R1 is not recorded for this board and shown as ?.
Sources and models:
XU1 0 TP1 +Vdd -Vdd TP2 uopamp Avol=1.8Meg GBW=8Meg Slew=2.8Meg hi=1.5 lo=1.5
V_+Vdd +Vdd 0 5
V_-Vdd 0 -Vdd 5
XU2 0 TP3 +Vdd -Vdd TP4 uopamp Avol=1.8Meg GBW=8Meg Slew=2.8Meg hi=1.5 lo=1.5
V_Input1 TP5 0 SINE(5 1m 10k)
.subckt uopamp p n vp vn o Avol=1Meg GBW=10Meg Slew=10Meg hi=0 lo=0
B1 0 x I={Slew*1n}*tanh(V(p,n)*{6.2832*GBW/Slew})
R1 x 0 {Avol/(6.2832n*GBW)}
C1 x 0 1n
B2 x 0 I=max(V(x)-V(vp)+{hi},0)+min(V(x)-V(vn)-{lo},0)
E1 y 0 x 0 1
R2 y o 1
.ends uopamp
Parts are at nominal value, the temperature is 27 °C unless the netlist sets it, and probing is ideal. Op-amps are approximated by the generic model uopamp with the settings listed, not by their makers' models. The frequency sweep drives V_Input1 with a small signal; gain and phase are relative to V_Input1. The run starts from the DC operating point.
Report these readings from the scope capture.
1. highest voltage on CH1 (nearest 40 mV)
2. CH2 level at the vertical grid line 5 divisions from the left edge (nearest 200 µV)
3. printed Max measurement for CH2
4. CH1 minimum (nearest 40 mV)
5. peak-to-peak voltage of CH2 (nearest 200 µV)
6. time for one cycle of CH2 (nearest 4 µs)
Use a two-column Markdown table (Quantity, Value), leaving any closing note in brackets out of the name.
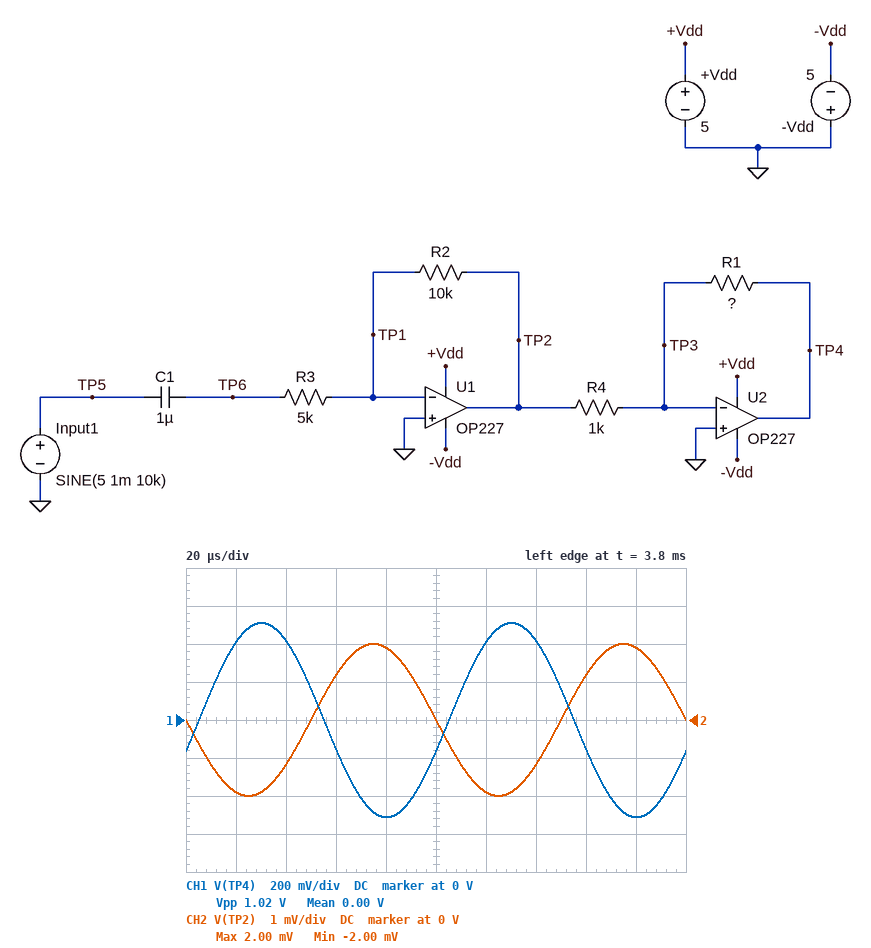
| Quantity | Value |
|---|---|
| highest voltage on CH1 | 520 mV |
| CH2 level at the vertical grid line 5 divisions from the left edge | 0 V |
| printed Max measurement for CH2 | 2.00 mV |
| CH1 minimum | -520 mV |
| peak-to-peak voltage of CH2 | 4.0 mV |
| time for one cycle of CH2 | 100 µs |
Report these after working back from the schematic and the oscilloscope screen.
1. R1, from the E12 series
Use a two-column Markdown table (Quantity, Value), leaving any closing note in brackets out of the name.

| Quantity | Value |
|---|---|
| R1, from the E12 series | 270 kΩ |
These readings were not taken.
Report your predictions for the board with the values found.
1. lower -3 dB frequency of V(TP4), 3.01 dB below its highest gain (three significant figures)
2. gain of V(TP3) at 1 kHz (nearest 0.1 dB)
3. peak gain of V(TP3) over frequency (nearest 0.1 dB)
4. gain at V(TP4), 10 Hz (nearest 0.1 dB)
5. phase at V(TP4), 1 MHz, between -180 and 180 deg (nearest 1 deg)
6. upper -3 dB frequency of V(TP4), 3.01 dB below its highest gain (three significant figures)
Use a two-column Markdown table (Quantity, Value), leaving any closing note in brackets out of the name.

| Quantity | Value |
|---|---|
| lower -3 dB frequency of V(TP4), 3.01 dB below its highest gain | 31.8 Hz |
| gain of V(TP3) at 1 kHz | -23.4 dB |
| peak gain of V(TP3) over frequency | 5.9 dB |
| gain at V(TP4), 10 Hz | 44.2 dB |
| phase at V(TP4), 1 MHz, between -180 and 180 deg | -109 deg |
| upper -3 dB frequency of V(TP4), 3.01 dB below its highest gain | 29.6 kHz |
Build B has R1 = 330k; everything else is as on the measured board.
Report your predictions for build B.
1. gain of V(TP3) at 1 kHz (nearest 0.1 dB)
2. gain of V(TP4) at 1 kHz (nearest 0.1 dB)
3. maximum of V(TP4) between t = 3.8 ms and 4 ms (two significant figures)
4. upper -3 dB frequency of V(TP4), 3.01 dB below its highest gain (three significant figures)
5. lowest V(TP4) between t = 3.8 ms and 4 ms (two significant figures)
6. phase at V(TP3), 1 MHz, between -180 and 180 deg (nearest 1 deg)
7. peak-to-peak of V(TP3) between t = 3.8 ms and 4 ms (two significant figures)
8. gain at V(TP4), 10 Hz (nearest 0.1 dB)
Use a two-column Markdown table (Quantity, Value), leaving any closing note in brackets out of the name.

| Quantity | Value |
|---|---|
| gain of V(TP3) at 1 kHz | -21.7 dB |
| gain of V(TP4) at 1 kHz | 56.4 dB |
| maximum of V(TP4) between t = 3.8 ms and 4 ms | 610 mV |
| upper -3 dB frequency of V(TP4), 3.01 dB below its highest gain | 24.2 kHz |
| lowest V(TP4) between t = 3.8 ms and 4 ms | -610 mV |
| phase at V(TP3), 1 MHz, between -180 and 180 deg | 161 deg |
| peak-to-peak of V(TP3) between t = 3.8 ms and 4 ms | 1.5 mV |
| gain at V(TP4), 10 Hz | 45.9 dB |
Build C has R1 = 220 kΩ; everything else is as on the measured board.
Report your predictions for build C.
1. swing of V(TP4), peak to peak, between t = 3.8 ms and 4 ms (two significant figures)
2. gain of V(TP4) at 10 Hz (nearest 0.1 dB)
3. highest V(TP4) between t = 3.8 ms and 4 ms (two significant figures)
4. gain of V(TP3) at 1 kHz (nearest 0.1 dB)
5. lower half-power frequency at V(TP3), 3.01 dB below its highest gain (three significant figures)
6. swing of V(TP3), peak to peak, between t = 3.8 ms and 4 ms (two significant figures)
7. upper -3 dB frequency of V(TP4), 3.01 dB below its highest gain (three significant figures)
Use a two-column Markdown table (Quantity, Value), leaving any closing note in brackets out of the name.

| Quantity | Value |
|---|---|
| swing of V(TP4), peak to peak, between t = 3.8 ms and 4 ms | 850 mV |
| gain of V(TP4) at 10 Hz | 42.4 dB |
| highest V(TP4) between t = 3.8 ms and 4 ms | 420 mV |
| gain of V(TP3) at 1 kHz | -25.2 dB |
| lower half-power frequency at V(TP3), 3.01 dB below its highest gain | 35.3 kHz |
| swing of V(TP3), peak to peak, between t = 3.8 ms and 4 ms | 1.1 mV |
| upper -3 dB frequency of V(TP4), 3.01 dB below its highest gain | 36.3 kHz |
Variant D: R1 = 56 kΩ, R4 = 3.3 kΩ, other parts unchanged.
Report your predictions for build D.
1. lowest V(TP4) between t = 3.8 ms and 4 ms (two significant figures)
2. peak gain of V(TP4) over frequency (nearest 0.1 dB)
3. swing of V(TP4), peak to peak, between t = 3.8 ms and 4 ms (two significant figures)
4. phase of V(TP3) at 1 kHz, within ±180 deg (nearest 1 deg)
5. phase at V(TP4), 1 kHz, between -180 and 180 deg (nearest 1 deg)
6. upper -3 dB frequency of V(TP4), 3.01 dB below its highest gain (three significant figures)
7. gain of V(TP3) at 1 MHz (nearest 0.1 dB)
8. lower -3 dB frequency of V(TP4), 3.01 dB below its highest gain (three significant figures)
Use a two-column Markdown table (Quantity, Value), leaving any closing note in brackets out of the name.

| Quantity | Value |
|---|---|
| lowest V(TP4) between t = 3.8 ms and 4 ms | -34 mV |
| peak gain of V(TP4) over frequency | 30.6 dB |
| swing of V(TP4), peak to peak, between t = 3.8 ms and 4 ms | 68 mV |
| phase of V(TP3) at 1 kHz, within ±180 deg | -89 deg |
| phase at V(TP4), 1 kHz, between -180 and 180 deg | 2 deg |
| upper -3 dB frequency of V(TP4), 3.01 dB below its highest gain | 434 kHz |
| gain of V(TP3) at 1 MHz | 4.2 dB |
| lower -3 dB frequency of V(TP4), 3.01 dB below its highest gain | 31.8 Hz |
